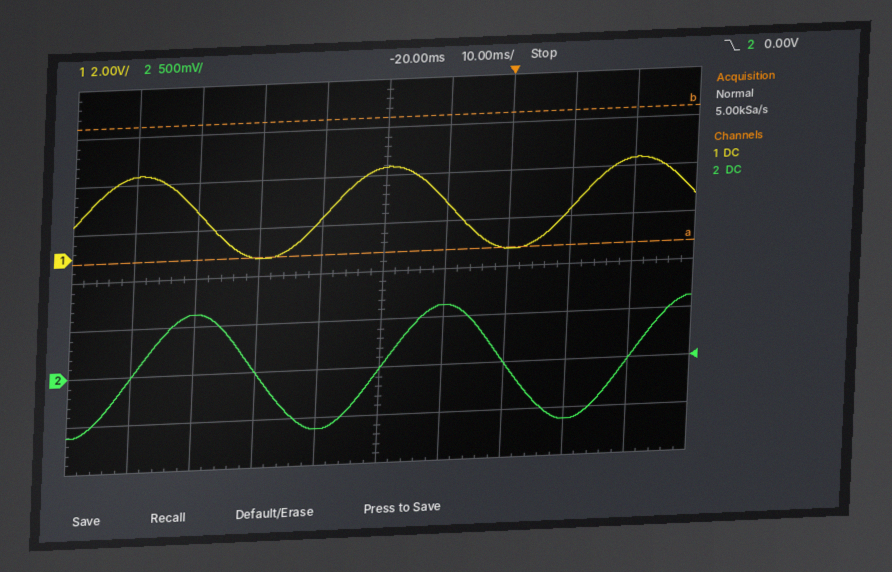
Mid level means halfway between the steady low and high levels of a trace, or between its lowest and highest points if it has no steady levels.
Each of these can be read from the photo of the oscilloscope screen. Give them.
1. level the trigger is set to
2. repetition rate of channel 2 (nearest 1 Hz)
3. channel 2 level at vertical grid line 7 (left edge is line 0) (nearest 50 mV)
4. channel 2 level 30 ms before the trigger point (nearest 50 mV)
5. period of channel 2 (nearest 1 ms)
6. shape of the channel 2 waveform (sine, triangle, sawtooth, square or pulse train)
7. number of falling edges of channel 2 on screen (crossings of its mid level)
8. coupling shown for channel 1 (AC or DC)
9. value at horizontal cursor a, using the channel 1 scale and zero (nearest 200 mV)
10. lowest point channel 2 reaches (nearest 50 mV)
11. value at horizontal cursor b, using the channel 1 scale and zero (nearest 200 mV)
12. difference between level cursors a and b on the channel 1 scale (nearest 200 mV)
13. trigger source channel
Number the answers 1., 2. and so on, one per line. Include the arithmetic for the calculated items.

1. 0.00 V
2. 1 / 40 ms ≈ 25 Hz
3. 0 mV
4. -600 mV
5. 40 ms
6. sine
7. 2
8. DC
9. -200 mV
10. -600 mV
11. 5.4 V
12. 5.6 V
13. channel 2
